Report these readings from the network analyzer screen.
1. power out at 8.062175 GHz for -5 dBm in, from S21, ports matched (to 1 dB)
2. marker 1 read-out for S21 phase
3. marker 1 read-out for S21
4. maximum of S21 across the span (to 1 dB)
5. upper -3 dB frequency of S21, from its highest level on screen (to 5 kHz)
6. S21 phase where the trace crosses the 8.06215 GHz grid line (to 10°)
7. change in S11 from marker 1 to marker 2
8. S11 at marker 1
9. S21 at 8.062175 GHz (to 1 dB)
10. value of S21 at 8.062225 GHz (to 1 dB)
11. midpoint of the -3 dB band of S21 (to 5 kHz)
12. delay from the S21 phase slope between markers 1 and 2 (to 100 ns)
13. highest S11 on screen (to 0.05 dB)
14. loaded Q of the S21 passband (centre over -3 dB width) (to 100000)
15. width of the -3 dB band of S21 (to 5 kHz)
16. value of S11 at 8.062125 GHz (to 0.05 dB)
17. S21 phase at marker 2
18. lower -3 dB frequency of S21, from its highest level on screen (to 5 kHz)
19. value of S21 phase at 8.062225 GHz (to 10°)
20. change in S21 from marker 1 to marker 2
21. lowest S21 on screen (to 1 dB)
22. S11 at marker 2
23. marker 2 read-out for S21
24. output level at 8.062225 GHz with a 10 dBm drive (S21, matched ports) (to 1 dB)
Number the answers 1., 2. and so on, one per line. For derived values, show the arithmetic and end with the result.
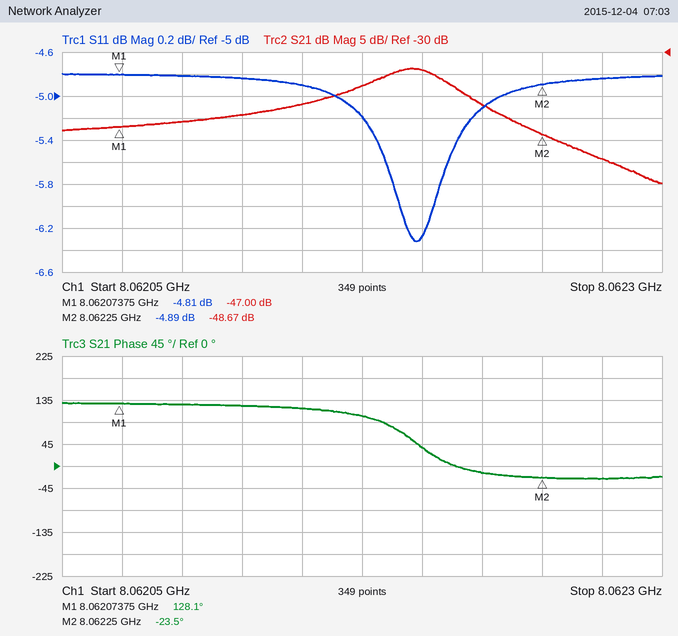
1. -5 dBm + (-38 dB) = -43 dBm
2. 128.1°
3. -47.00 dB
4. -34 dB
5. 8.062210 GHz
6. 120°
7. -4.89 − (-4.81) = -0.08 dB
8. -4.81 dB
9. -38 dB
10. -42 dB
11. 8.062195 GHz
12. −(-23.5° − (128.1°))/(360° × 176.25 kHz) ≈ 2.4 µs
13. -4.80 dB
14. 8.0622 GHz / 30 kHz ≈ 268740, so 300000 to the nearest 100000
15. 8.062210 GHz − 8.062180 GHz = 30 kHz
16. -4.85 dB
17. -23.5°
18. 8.062180 GHz
19. -10°
20. -48.67 − (-47) = -1.67 dB
21. -60 dB
22. -4.89 dB
23. -48.67 dB
24. 10 dBm + (-42 dB) = -32 dBm
